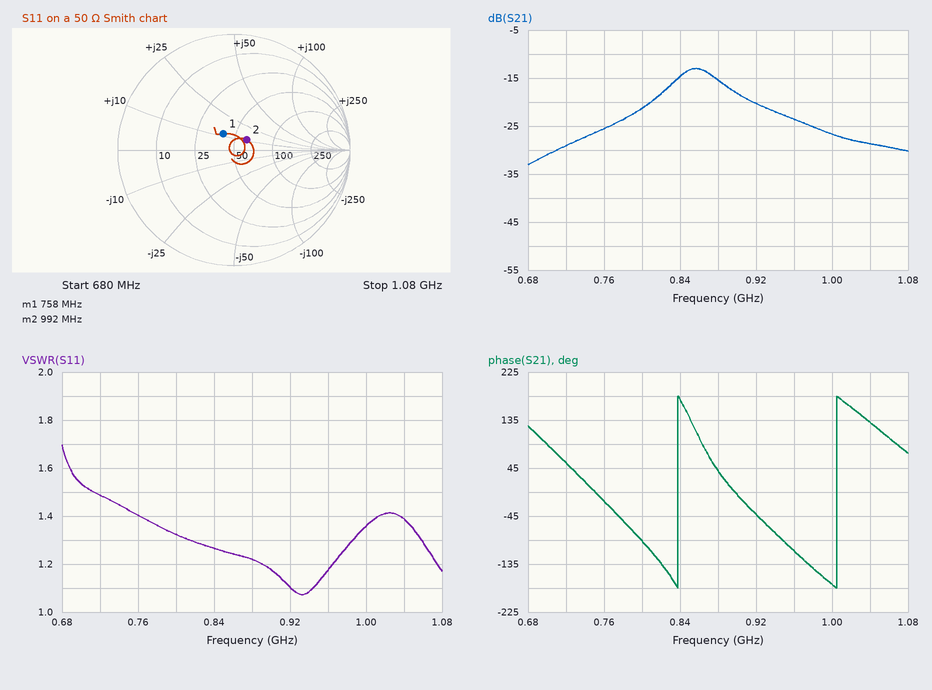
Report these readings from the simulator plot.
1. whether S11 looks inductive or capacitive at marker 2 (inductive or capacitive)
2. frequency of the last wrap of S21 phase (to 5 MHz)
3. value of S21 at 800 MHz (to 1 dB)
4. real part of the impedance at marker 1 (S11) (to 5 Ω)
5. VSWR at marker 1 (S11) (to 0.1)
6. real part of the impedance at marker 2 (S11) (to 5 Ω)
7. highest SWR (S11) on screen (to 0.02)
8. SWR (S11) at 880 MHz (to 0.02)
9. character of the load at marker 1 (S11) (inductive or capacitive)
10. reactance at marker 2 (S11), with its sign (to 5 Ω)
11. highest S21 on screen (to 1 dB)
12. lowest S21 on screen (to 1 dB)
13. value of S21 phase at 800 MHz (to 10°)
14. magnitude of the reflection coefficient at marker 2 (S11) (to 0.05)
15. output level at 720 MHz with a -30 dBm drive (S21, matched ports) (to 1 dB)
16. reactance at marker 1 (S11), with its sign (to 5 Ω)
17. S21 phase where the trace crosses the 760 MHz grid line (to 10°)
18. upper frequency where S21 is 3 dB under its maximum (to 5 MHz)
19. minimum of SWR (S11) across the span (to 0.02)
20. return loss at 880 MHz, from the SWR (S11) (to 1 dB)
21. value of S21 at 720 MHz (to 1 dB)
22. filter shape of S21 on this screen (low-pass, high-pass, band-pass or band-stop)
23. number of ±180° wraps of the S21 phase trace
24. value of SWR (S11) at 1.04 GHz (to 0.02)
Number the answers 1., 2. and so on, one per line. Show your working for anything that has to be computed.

1. inductive
2. 1.005 GHz
3. -21 dB
4. 40 Ω
5. 1.4
6. 60 Ω
7. 1.70
8. 1.22
9. inductive
10. +10 Ω
11. -13 dB
12. -33 dB
13. -90°
14. 0.15
15. -30 dBm + (-29 dB) = -59 dBm
16. +10 Ω
17. -20°
18. 885 MHz
19. 1.08
20. −20 log10((1.22 − 1)/(1.22 + 1)) ≈ 20 dB
21. -29 dB
22. band-pass
23. 2
24. 1.38
